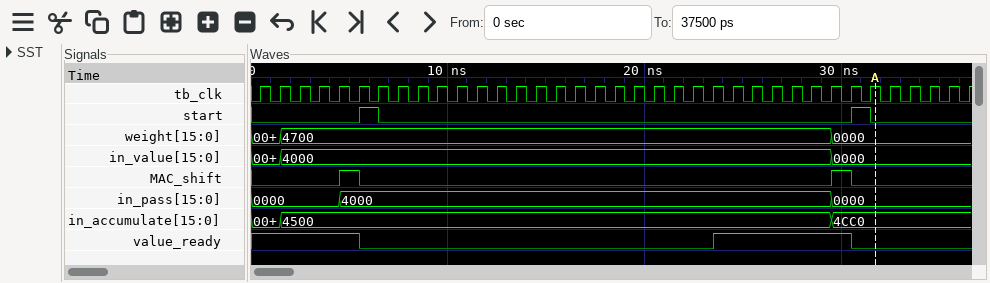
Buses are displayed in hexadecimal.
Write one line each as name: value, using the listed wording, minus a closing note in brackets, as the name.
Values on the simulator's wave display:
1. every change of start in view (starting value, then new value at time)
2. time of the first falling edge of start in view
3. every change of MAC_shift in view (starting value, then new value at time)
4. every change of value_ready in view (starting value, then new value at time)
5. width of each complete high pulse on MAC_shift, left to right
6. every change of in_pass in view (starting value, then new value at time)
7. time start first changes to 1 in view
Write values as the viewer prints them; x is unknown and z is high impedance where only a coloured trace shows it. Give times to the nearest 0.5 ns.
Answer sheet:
every change of start in view: 0, 1 at 5.5 ns, 0 at 6.5 ns, 1 at 30.5 ns, 0 at 31.5 ns
time of the first falling edge of start in view: 6.5 ns
every change of MAC_shift in view: 0, 1 at 4.5 ns, 0 at 5.5 ns, 1 at 29.5 ns, 0 at 30.5 ns
every change of value_ready in view: 1, 0 at 5.5 ns, 1 at 23.5 ns, 0 at 30.5 ns
width of each complete high pulse on MAC_shift, left to right: 1 ns, 1 ns
every change of in_pass in view: 0000, 4000 at 4.5 ns, 0000 at 29.5 ns
time start first changes to 1 in view: 5.5 ns
